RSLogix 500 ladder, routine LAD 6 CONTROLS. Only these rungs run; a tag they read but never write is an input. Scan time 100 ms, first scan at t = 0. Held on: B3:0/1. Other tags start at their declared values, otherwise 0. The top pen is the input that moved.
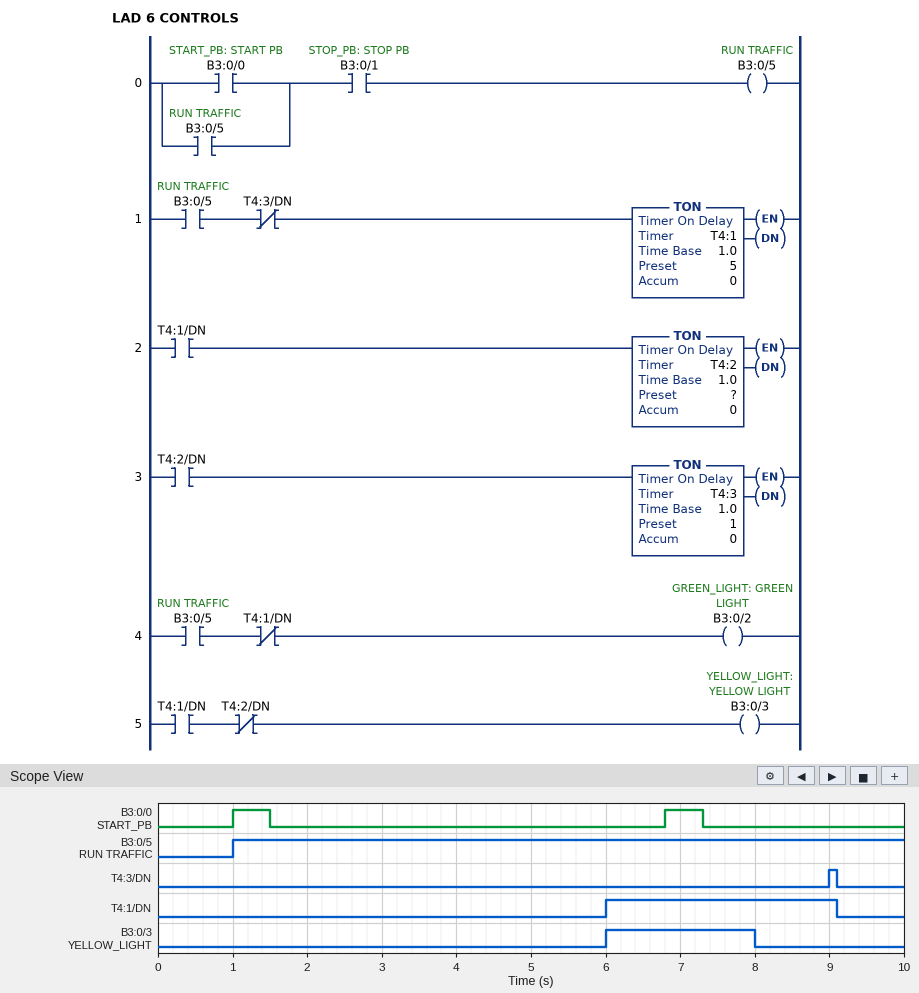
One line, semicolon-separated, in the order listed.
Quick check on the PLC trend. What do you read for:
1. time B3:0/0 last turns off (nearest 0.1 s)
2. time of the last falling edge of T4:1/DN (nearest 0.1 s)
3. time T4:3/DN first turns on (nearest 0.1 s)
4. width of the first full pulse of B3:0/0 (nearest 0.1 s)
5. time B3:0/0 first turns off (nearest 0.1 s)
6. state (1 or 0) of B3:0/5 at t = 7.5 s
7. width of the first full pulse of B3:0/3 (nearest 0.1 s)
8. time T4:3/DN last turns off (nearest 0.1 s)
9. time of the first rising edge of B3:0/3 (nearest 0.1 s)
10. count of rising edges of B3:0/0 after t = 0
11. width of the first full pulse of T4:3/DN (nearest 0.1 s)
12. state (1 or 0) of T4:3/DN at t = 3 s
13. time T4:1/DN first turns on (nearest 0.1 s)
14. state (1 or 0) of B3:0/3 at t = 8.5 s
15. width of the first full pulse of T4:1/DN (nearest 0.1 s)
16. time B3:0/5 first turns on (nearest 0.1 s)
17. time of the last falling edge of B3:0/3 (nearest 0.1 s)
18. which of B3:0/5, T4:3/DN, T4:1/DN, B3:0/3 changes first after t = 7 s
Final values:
7.3 s; 9.1 s; 9.0 s; 0.5 s; 1.5 s; 1; 2.0 s; 9.1 s; 6.0 s; 2; 0.1 s; 0; 6.0 s; 0; 3.1 s; 1.0 s; 8.0 s; B3:0/3
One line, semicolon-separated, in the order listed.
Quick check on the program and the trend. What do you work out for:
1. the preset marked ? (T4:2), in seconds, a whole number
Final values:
2 s
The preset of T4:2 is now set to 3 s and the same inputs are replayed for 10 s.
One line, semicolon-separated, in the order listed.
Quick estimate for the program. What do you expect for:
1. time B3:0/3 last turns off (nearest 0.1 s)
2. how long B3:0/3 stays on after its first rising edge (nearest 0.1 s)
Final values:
9.0 s; 3.0 s
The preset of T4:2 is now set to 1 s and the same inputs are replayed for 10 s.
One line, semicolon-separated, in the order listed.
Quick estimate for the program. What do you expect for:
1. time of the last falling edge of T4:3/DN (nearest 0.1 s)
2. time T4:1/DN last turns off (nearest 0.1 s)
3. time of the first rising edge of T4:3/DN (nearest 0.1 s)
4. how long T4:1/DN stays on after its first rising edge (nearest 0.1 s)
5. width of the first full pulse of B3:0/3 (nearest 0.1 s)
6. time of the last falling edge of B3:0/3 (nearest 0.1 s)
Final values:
8.1 s; 8.1 s; 8.0 s; 2.1 s; 1.0 s; 7.0 s
